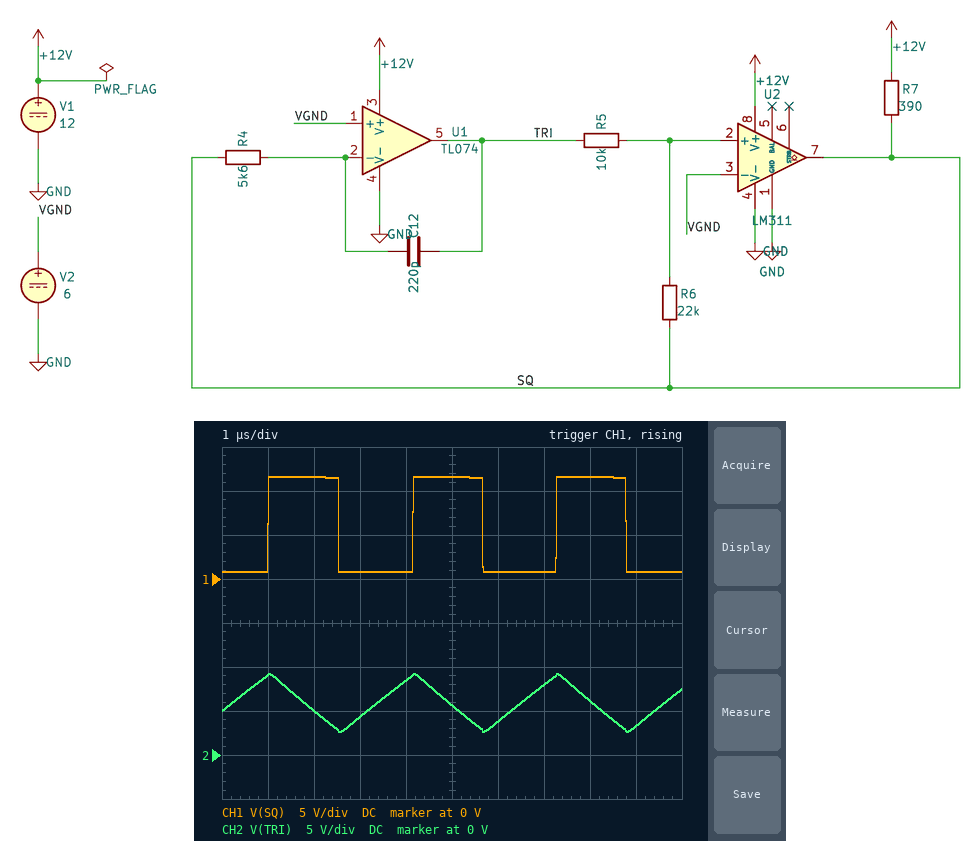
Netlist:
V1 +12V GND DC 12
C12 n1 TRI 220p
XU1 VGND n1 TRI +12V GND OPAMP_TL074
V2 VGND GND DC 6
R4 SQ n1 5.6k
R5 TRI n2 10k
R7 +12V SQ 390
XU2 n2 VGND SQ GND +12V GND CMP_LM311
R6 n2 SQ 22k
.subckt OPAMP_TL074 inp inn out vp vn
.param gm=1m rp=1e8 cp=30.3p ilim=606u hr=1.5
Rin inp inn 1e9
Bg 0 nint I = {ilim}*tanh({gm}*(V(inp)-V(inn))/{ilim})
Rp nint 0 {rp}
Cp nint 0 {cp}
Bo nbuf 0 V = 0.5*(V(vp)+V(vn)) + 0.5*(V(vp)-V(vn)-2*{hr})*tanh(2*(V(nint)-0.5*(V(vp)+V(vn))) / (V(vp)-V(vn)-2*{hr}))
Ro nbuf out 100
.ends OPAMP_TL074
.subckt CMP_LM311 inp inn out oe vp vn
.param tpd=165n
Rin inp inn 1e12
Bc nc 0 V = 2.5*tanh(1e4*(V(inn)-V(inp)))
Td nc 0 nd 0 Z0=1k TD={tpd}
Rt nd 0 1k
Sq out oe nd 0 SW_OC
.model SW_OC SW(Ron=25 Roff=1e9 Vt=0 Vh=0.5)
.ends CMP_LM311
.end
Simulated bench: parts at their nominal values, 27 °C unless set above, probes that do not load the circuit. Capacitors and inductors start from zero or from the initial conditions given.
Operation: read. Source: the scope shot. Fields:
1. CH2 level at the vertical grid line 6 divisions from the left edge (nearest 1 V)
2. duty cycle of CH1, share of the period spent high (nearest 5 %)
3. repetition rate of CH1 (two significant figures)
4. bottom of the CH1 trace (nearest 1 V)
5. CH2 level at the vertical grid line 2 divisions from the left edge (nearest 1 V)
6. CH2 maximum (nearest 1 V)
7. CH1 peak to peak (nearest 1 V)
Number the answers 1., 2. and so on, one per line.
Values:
1. 4 V
2. 50 %
3. 320 kHz
4. 1 V
5. 5 V
6. 9 V
7. 11 V
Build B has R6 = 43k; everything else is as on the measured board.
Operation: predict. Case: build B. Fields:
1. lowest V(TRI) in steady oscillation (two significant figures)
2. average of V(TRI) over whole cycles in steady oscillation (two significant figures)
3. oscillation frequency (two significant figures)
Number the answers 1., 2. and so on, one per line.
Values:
1. 3.8 V
2. 5.9 V
3. 510 kHz
